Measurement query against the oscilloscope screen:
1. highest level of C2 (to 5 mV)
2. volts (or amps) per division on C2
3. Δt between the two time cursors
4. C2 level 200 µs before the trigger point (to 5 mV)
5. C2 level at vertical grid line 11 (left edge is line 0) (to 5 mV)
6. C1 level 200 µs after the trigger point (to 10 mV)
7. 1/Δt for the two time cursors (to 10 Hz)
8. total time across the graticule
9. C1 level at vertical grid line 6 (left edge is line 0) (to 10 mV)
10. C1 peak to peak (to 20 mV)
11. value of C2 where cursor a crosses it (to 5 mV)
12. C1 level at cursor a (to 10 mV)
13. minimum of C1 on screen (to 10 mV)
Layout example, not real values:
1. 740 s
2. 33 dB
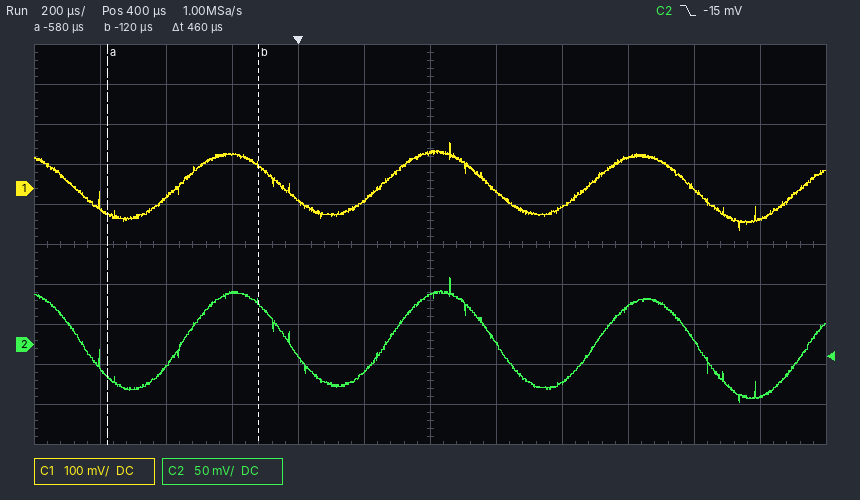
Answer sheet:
1. 85 mV
2. 50 mV
3. 460 µs
4. 65 mV
5. -65 mV
6. -30 mV
7. 2.17 kHz
8. 2.4 ms
9. 90 mV
10. 220 mV
11. -40 mV
12. -60 mV
13. -100 mV
